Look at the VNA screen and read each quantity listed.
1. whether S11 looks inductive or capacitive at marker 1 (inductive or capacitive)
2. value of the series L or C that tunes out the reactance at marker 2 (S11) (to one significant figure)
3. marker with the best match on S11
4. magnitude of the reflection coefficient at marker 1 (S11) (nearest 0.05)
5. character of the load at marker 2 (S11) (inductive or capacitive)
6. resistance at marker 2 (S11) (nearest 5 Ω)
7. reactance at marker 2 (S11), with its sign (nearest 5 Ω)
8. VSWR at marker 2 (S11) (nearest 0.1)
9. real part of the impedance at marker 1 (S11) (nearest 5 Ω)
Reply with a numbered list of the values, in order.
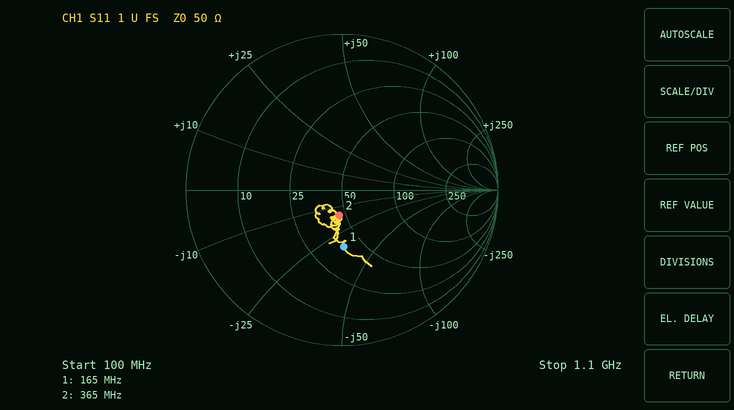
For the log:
1. capacitive
2. 7 nH
3. marker 2
4. 0.35
5. capacitive
6. 45 Ω
7. -15 Ω
8. 1.4
9. 40 Ω
